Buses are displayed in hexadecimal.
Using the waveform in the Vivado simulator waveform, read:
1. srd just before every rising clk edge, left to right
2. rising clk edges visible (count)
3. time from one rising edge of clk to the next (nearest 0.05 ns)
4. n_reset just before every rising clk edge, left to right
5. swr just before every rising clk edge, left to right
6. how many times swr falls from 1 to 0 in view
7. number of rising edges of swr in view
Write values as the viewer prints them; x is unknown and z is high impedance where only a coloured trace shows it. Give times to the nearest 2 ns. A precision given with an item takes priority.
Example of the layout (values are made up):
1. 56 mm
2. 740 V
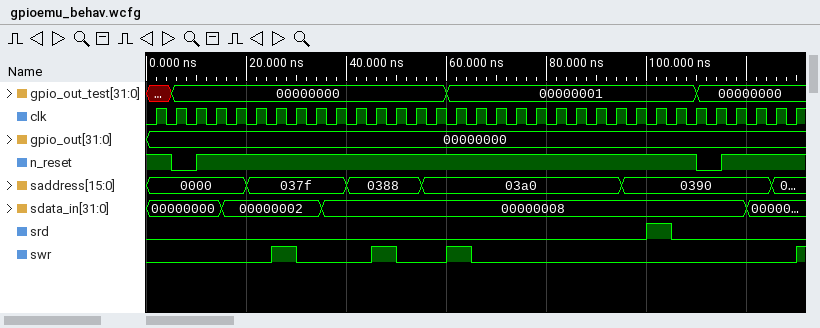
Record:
1. 0 0 0 0 0 0 0 0 0 0 0 0 0 0 0 0 0 0 0 0 0 0 0 0 0 1 0 0 0 0 0 0 0
2. 33
3. 4 ns
4. 1 0 0 1 1 1 1 1 1 1 1 1 1 1 1 1 1 1 1 1 1 1 1 1 1 1 1 1 0 1 1 1 1
5. 0 0 0 0 0 0 1 1 0 0 0 1 1 0 0 1 0 0 0 0 0 0 0 0 0 0 0 0 0 0 0 0 0
6. 3
7. 4
